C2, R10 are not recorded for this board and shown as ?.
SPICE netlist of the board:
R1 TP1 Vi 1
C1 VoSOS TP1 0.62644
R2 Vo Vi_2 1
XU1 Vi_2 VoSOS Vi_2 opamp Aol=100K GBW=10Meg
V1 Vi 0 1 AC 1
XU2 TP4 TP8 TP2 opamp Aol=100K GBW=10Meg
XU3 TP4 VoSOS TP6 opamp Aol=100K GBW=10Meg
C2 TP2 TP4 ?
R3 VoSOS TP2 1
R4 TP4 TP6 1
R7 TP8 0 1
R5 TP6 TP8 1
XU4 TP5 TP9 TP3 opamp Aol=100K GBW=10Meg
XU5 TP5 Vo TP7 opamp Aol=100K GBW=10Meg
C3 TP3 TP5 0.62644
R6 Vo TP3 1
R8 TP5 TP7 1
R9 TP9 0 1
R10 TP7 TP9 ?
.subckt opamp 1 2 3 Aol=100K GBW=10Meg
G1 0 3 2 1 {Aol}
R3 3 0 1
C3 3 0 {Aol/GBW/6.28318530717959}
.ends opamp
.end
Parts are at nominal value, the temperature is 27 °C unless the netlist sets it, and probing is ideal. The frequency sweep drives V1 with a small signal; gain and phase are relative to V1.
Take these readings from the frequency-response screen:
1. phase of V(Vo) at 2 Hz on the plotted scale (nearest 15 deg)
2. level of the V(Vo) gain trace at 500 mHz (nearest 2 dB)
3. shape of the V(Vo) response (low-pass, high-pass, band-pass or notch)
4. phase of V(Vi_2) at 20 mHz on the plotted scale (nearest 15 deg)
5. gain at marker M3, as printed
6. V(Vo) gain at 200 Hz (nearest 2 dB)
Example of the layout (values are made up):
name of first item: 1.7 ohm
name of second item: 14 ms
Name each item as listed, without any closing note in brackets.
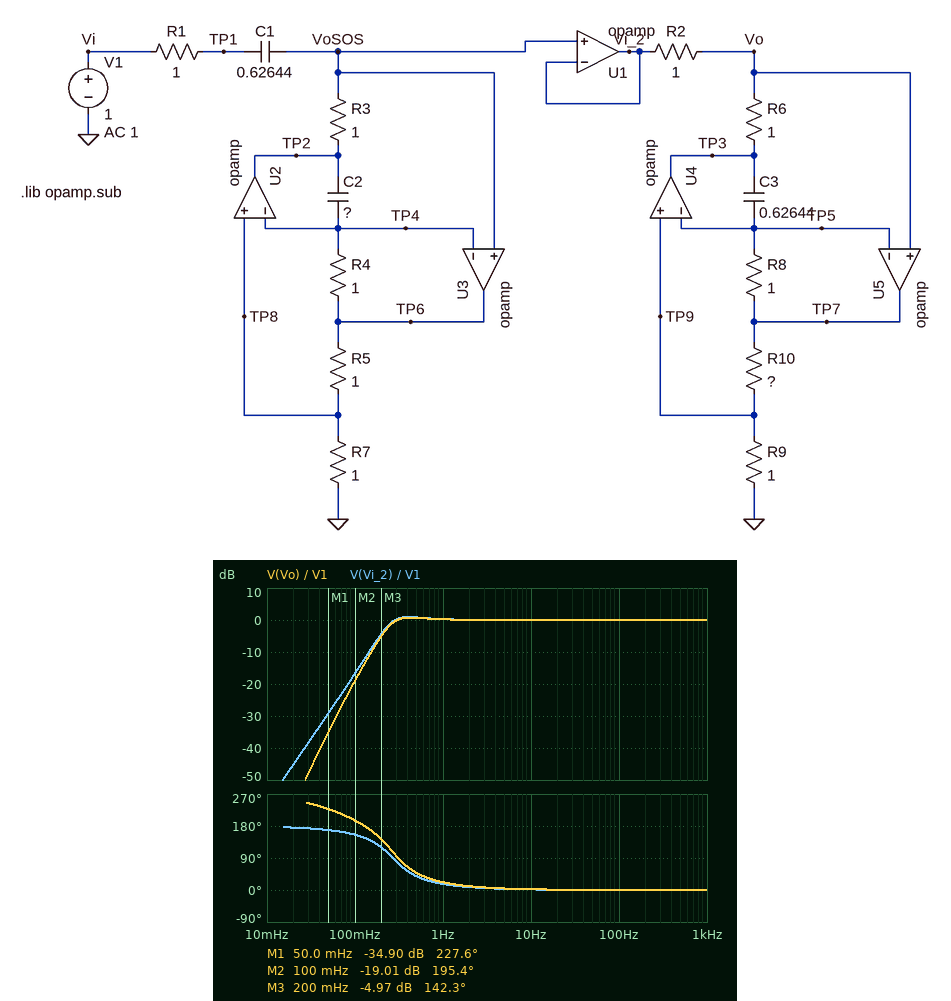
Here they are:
phase of V(Vo) at 2 Hz on the plotted scale: 15 deg
level of the V(Vo) gain trace at 500 mHz: 0 dB
shape of the V(Vo) response: high-pass
phase of V(Vi_2) at 20 mHz on the plotted scale: 180 deg
gain at marker M3, as printed: -4.97 dB
V(Vo) gain at 200 Hz: 0 dB
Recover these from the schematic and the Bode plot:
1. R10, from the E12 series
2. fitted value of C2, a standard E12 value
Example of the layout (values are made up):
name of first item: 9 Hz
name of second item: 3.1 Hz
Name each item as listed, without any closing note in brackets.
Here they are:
R10, from the E12 series: 0.33 Ω
fitted value of C2, a standard E12 value: 560 mF
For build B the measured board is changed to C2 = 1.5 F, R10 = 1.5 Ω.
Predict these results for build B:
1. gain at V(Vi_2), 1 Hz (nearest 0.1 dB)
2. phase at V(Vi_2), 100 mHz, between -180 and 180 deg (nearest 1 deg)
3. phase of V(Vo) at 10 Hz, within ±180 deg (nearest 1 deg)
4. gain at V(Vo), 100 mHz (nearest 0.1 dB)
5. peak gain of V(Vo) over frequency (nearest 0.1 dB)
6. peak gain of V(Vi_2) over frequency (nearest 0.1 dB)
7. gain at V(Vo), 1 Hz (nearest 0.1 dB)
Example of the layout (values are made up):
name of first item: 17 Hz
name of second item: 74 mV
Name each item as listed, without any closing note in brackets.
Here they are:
gain at V(Vi_2), 1 Hz: 0.2 dB
phase at V(Vi_2), 100 mHz, between -180 and 180 deg: 148 deg
phase of V(Vo) at 10 Hz, within ±180 deg: 3 deg
gain at V(Vo), 100 mHz: -17.9 dB
peak gain of V(Vo) over frequency: 0 dB
peak gain of V(Vi_2) over frequency: 4.3 dB
gain at V(Vo), 1 Hz: -0.4 dB
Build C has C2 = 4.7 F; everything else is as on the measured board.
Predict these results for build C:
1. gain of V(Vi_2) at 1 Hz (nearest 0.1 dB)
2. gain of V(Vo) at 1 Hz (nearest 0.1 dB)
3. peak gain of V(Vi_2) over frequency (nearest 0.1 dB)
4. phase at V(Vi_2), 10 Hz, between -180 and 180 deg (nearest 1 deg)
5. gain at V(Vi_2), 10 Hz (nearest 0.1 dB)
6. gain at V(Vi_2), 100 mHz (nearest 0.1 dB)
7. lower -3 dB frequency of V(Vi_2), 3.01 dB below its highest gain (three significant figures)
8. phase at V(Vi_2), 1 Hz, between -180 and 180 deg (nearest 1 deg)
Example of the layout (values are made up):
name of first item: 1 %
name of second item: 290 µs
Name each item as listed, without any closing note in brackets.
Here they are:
gain of V(Vi_2) at 1 Hz: 0.1 dB
gain of V(Vo) at 1 Hz: 0 dB
peak gain of V(Vi_2) over frequency: 8.9 dB
phase at V(Vi_2), 10 Hz, between -180 and 180 deg: 0 deg
gain at V(Vi_2), 10 Hz: 0 dB
gain at V(Vi_2), 100 mHz: 8.7 dB
lower -3 dB frequency of V(Vi_2), 3.01 dB below its highest gain: 81.6 mHz
phase at V(Vi_2), 1 Hz, between -180 and 180 deg: 2 deg
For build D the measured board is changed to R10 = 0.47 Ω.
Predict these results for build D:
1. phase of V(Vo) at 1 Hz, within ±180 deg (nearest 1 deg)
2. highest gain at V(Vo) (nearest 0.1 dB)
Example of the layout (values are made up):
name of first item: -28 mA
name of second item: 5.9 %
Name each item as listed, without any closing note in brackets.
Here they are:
phase of V(Vo) at 1 Hz, within ±180 deg: 24 deg
highest gain at V(Vo): 0.6 dB
